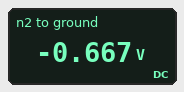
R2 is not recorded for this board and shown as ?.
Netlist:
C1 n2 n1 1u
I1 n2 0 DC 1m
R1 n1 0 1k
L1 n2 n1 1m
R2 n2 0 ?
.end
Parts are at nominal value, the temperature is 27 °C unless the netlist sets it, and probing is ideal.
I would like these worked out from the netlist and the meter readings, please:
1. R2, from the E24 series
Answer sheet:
2 kΩ
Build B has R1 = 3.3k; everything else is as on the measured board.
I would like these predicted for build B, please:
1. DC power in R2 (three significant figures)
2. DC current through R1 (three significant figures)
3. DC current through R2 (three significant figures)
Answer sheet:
775 µW
377 µA
623 µA
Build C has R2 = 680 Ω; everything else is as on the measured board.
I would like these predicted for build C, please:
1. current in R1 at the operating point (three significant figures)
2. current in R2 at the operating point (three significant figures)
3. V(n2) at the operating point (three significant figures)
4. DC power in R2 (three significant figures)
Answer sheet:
405 µA
595 µA
-405 mV
241 µW
